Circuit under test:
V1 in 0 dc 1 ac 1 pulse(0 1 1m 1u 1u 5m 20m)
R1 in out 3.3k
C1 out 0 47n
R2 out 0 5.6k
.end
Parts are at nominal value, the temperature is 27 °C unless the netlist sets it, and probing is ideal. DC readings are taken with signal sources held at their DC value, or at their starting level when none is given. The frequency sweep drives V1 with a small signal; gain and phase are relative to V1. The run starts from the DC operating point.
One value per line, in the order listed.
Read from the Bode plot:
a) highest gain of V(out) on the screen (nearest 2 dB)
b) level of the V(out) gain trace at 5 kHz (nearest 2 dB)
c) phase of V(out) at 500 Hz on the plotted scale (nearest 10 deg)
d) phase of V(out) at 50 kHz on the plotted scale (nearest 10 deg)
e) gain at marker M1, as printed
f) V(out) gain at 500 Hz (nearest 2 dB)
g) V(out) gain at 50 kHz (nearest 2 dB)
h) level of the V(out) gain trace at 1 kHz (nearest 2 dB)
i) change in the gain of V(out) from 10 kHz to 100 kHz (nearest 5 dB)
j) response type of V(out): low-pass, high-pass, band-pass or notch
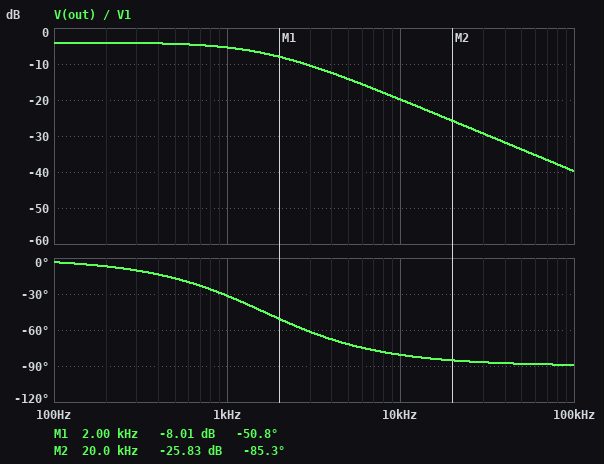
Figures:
-4 dB
-14 dB
-20 deg
-90 deg
-8.01 dB
-4 dB
-34 dB
-6 dB
-20 dB
low-pass
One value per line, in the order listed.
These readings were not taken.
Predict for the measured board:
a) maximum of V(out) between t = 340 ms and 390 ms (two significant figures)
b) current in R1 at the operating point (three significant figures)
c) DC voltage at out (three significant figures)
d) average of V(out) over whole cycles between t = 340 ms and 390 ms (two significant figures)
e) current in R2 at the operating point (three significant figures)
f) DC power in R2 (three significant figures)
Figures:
630 mV
112 µA
629 mV
160 mV
112 µA
70.7 µW
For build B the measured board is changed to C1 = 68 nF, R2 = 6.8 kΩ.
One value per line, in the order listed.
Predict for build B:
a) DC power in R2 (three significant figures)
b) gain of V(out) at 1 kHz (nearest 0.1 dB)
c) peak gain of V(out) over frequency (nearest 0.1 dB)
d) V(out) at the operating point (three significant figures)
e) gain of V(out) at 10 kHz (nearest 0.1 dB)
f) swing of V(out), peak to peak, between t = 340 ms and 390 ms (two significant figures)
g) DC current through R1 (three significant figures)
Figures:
66.7 µW
-6.2 dB
-3.4 dB
673 mV
-23.0 dB
670 mV
99.0 µA
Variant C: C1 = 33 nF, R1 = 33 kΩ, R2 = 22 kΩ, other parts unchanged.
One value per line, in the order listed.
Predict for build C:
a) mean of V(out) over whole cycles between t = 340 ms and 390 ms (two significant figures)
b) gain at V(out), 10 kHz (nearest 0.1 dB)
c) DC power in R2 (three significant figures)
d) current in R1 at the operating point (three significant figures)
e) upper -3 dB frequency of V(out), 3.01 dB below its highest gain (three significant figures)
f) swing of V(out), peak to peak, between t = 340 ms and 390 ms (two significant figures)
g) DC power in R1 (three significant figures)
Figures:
100 mV
-36.7 dB
7.27 µW
18.2 µA
365 Hz
400 mV
10.9 µW
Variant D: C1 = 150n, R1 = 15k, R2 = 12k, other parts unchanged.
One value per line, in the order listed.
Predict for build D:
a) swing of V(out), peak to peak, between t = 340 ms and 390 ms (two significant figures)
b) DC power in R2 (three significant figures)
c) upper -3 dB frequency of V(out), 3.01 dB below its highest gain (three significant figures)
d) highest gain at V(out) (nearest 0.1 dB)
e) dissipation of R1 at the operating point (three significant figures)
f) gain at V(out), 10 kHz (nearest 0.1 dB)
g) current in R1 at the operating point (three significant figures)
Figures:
440 mV
16.5 µW
159 Hz
-7.0 dB
20.6 µW
-43.0 dB
37.0 µA
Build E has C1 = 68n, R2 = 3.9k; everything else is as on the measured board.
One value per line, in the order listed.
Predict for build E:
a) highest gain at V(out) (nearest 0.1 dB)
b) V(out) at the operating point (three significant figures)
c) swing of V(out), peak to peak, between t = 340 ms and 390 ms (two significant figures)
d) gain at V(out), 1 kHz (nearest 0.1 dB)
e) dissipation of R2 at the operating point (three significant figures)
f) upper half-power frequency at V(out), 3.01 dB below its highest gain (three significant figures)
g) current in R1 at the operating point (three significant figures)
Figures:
-5.3 dB
542 mV
540 mV
-7.3 dB
75.2 µW
1.31 kHz
139 µA
